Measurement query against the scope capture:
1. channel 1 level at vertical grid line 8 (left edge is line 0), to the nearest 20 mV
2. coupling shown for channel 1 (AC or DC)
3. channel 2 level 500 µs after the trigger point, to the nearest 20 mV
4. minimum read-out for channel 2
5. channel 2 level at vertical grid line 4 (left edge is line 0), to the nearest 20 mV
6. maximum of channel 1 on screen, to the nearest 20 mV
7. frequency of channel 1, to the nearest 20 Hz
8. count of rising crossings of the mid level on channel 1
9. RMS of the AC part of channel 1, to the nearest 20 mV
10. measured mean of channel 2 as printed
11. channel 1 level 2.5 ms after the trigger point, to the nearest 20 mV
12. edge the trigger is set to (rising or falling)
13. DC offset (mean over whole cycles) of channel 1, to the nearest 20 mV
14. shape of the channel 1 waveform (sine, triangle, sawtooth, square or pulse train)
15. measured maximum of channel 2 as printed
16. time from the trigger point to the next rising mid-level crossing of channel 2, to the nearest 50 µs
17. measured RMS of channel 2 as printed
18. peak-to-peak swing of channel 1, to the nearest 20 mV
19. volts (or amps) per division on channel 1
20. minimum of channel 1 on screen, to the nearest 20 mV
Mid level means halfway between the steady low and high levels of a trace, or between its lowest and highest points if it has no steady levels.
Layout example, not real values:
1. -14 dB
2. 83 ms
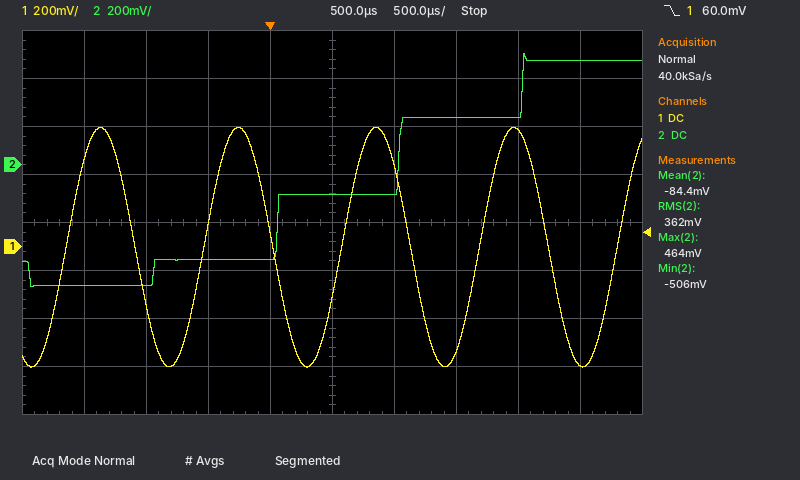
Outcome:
1. 480 mV
2. DC
3. -120 mV
4. -506 mV
5. -400 mV
6. 500 mV
7. 900 Hz
8. 5
9. 360 mV
10. -84.4 mV
11. -500 mV
12. falling
13. 0 mV
14. sine
15. 464 mV
16. 1.05 ms
17. 362 mV
18. 1.00 V
19. 200 mV
20. -500 mV
